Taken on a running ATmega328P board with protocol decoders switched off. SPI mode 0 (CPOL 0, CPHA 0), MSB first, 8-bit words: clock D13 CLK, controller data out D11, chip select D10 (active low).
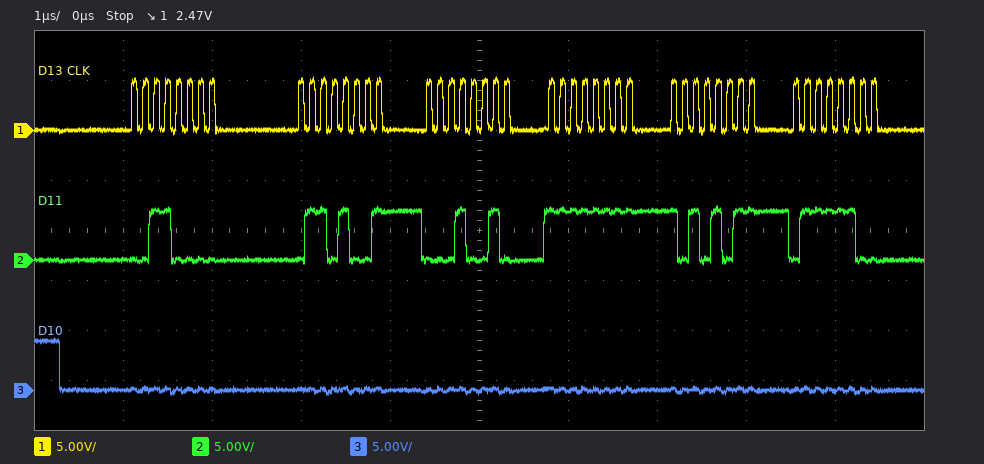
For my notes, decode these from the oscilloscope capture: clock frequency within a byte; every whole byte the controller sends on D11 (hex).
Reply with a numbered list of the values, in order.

1. 8 MHz
2. 0x30 0x69 0x12 0xFF 0xAB 0x7C
